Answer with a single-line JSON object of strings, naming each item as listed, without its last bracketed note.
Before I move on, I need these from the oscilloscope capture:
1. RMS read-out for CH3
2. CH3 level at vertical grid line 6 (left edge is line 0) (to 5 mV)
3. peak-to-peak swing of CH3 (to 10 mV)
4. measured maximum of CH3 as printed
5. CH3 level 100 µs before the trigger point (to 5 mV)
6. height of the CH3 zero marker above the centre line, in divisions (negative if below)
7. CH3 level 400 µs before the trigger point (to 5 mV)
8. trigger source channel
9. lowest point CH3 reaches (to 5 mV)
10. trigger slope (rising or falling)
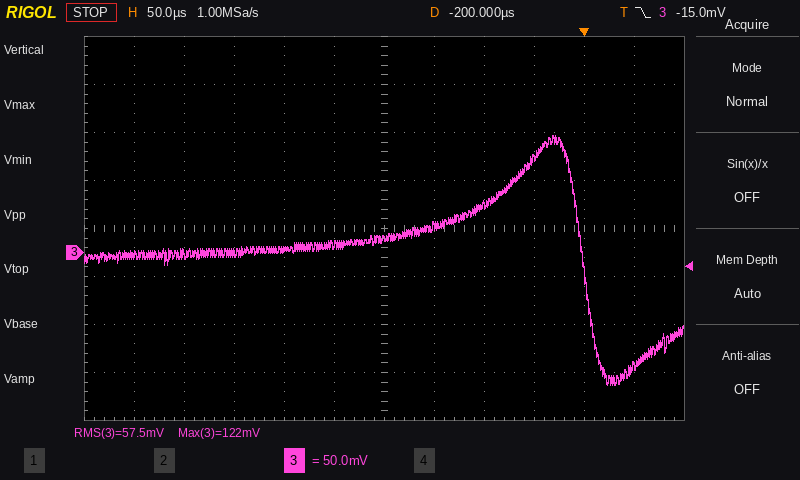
{"RMS read-out for CH3": "57.5 mV", "CH3 level at vertical grid line 6 (left edge is line 0)": "15 mV", "peak-to-peak swing of CH3": "260 mV", "measured maximum of CH3 as printed": "122 mV", "CH3 level 100 µs before the trigger point": "50 mV", "height of the CH3 zero marker above the centre line, in divisions": "-0.5 div", "CH3 level 400 µs before the trigger point": "0 mV", "trigger source channel": "CH3", "lowest point CH3 reaches": "-140 mV", "trigger slope": "falling"}
